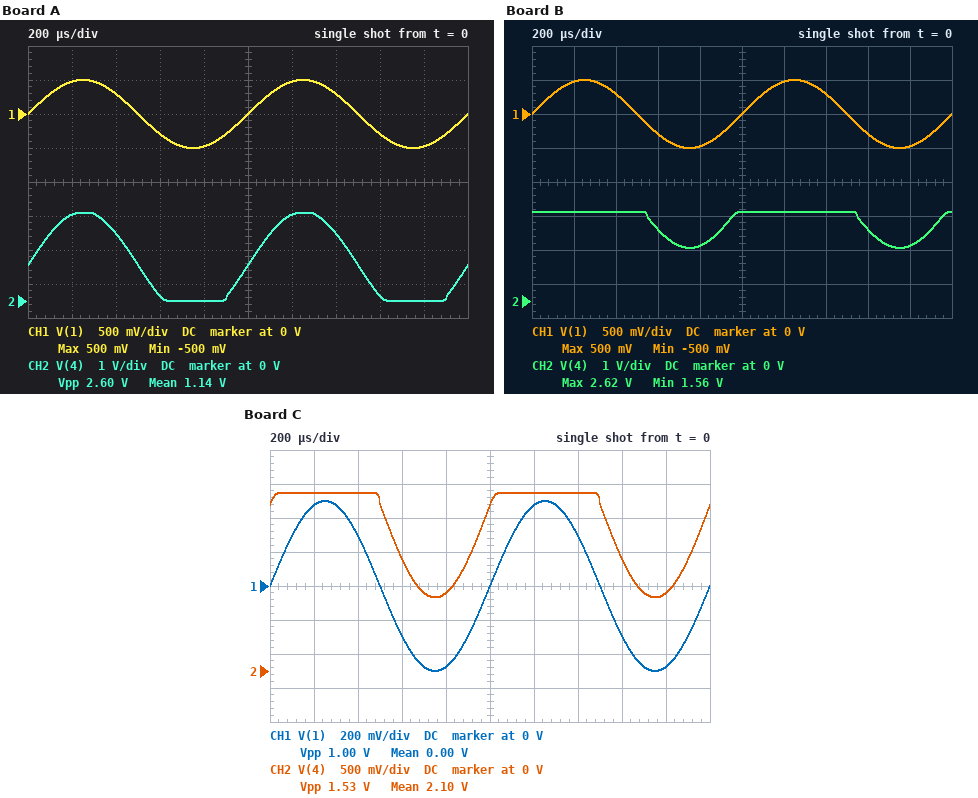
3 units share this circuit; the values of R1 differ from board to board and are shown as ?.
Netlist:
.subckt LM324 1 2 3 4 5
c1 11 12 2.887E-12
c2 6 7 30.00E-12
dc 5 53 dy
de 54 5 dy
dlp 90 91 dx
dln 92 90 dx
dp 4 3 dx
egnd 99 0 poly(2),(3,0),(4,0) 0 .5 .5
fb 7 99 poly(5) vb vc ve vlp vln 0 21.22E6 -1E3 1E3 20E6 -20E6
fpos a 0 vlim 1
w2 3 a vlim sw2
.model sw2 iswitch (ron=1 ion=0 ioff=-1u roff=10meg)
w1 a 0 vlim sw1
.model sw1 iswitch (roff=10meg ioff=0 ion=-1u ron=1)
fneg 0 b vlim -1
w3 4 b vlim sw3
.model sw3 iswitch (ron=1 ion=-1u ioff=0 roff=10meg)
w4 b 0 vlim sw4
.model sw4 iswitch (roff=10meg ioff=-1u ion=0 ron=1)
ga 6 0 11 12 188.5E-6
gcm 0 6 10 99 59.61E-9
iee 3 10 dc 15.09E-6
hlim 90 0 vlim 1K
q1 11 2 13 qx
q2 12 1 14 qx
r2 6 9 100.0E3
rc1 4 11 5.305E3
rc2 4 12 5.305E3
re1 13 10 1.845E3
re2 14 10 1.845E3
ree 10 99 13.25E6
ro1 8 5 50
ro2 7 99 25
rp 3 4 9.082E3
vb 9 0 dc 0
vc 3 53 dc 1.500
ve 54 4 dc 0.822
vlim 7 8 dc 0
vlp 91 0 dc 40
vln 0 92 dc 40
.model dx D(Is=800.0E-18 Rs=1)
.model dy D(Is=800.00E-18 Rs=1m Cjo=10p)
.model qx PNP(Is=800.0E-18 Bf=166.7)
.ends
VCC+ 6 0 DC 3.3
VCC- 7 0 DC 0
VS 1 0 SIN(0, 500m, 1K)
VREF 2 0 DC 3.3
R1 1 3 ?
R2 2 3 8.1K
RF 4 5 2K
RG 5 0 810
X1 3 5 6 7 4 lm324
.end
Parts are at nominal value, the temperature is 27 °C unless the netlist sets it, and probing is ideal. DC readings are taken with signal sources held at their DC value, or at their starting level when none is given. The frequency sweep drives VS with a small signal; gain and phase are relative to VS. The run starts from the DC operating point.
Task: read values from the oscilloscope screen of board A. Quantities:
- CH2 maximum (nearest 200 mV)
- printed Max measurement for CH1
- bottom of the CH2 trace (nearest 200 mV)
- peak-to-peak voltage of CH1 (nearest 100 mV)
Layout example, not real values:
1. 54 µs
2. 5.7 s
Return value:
1. 2.6 V
2. 500 mV
3. 0 V
4. 1.0 V
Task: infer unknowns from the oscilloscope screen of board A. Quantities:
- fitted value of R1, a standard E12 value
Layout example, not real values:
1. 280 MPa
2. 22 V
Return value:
1. 820 Ω
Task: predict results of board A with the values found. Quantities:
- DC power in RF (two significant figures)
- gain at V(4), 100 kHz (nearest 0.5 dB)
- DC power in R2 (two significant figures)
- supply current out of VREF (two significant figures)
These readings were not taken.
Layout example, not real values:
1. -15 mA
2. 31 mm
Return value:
1. 280 µW
2. 9.5 dB
3. 1.1 mW
4. 370 µA
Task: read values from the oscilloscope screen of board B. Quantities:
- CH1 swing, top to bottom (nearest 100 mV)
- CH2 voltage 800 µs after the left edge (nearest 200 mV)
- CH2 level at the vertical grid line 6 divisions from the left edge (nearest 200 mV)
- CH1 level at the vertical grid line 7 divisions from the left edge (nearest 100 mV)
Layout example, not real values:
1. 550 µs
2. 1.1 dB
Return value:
1. 1.0 V
2. 1.6 V
3. 2.6 V
4. 300 mV
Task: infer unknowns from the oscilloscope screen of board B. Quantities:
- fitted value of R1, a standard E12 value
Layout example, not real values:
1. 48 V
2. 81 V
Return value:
1. 2.7 kΩ
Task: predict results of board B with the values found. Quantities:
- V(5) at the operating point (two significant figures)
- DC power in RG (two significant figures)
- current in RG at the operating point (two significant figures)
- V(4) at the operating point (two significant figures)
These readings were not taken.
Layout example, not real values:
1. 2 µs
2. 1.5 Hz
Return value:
1. 750 mV
2. 700 µW
3. 930 µA
4. 2.6 V
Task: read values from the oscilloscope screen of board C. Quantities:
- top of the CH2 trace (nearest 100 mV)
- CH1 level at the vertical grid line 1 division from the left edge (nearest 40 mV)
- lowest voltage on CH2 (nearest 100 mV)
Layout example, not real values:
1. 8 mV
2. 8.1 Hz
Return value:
1. 2.6 V
2. 480 mV
3. 1.1 V
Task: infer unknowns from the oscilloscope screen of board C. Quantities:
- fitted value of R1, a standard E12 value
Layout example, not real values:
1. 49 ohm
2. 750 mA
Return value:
1. 2.2 kΩ
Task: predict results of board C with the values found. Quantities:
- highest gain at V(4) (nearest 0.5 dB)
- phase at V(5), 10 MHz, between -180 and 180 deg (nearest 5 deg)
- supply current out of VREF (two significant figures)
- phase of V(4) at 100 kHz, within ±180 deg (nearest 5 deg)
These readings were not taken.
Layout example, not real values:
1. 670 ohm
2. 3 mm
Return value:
1. 8.5 dB
2. -155 deg
3. 320 µA
4. -20 deg
